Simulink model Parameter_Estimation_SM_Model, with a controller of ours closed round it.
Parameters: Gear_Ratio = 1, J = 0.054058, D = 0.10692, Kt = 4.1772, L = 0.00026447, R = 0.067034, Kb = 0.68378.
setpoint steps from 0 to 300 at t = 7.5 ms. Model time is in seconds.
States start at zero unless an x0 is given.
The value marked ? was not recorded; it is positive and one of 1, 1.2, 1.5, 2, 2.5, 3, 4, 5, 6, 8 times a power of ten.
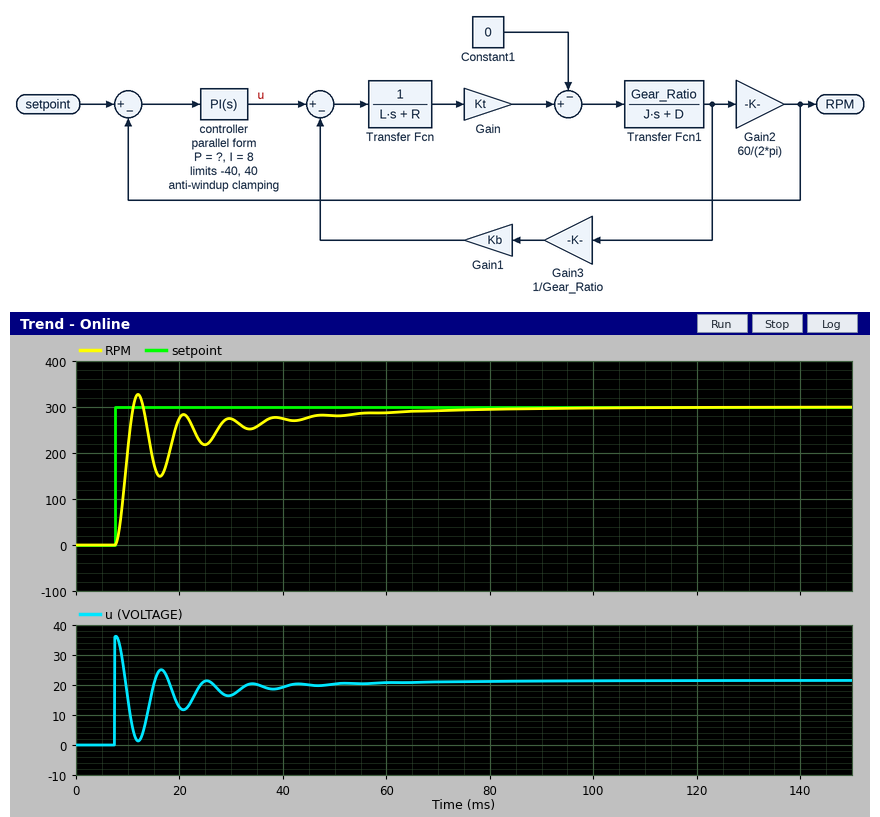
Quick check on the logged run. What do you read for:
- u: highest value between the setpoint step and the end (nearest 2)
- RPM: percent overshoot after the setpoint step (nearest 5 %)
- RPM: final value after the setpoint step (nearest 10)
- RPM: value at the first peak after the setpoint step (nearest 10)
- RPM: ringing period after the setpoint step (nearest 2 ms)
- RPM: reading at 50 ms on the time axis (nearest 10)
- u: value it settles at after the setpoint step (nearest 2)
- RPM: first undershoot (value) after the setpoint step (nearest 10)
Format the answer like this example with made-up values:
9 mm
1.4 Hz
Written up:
36
10 %
300
330
8 ms
280
22
150
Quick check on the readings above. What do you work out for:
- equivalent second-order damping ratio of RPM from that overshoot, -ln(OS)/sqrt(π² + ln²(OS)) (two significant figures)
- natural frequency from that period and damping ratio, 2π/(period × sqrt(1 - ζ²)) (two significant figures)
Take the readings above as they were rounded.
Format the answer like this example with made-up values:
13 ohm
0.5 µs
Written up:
0.59
0.97 rad/ms
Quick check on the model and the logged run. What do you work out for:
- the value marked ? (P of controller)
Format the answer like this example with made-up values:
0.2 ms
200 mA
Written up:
0.12
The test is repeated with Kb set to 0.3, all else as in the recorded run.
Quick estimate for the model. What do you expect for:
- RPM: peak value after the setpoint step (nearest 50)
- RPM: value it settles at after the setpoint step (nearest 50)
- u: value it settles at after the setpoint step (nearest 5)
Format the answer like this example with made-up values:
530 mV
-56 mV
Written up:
400
300
10
